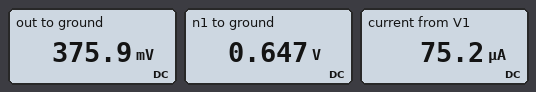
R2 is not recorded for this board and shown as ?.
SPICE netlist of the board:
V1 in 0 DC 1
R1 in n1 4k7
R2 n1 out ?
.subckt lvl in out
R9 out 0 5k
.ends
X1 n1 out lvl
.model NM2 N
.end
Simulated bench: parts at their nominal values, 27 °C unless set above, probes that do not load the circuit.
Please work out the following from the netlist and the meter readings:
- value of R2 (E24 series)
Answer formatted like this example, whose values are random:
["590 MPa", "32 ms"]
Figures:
["3.6 kΩ"]
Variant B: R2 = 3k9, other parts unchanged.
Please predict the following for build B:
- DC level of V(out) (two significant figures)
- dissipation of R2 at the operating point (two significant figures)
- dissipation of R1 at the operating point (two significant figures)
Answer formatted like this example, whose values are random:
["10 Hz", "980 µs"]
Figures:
["370 mV", "21 µW", "25 µW"]
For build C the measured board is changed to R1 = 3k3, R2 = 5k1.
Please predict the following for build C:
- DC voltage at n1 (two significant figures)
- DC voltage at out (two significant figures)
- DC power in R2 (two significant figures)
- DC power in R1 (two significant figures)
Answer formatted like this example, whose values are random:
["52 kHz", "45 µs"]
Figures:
["750 mV", "370 mV", "28 µW", "18 µW"]
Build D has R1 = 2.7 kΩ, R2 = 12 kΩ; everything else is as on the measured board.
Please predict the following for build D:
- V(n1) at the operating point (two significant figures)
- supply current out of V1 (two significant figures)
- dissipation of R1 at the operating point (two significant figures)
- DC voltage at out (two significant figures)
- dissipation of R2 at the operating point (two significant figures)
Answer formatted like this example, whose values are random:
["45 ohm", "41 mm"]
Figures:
["860 mV", "51 µA", "7.0 µW", "250 mV", "31 µW"]
